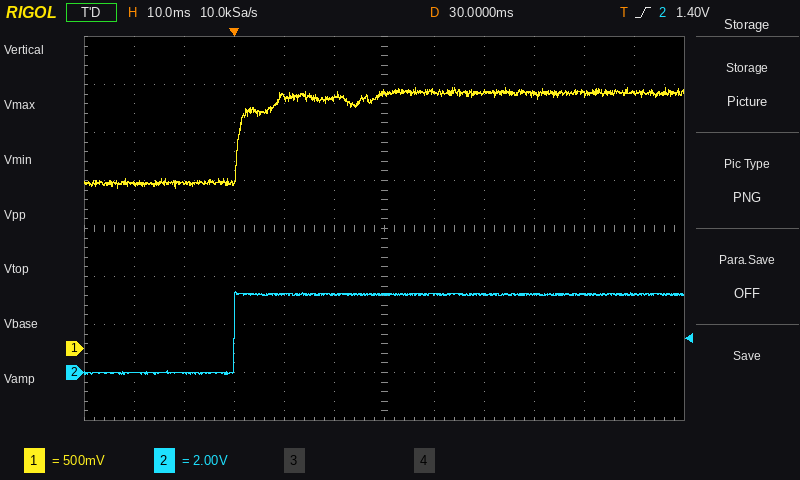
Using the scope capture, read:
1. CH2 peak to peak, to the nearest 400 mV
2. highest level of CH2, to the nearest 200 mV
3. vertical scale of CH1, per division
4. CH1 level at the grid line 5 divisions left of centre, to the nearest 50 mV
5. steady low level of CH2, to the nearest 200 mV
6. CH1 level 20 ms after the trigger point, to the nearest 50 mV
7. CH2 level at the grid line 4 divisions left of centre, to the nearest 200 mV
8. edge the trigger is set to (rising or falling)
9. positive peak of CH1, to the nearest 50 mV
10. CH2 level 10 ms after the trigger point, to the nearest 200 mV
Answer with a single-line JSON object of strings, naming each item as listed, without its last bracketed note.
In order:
{"CH2 peak to peak, to the nearest 400 mV": "3.6 V", "highest level of CH2, to the nearest 200 mV": "3.4 V", "vertical scale of CH1, per division": "500 mV", "CH1 level at the grid line 5 divisions left of centre, to the nearest 50 mV": "1.70 V", "steady low level of CH2, to the nearest 200 mV": "0.0 V", "CH1 level 20 ms after the trigger point, to the nearest 50 mV": "2.60 V", "CH2 level at the grid line 4 divisions left of centre, to the nearest 200 mV": "0.0 V", "edge the trigger is set to": "rising", "positive peak of CH1, to the nearest 50 mV": "2.70 V", "CH2 level 10 ms after the trigger point, to the nearest 200 mV": "3.2 V"}
